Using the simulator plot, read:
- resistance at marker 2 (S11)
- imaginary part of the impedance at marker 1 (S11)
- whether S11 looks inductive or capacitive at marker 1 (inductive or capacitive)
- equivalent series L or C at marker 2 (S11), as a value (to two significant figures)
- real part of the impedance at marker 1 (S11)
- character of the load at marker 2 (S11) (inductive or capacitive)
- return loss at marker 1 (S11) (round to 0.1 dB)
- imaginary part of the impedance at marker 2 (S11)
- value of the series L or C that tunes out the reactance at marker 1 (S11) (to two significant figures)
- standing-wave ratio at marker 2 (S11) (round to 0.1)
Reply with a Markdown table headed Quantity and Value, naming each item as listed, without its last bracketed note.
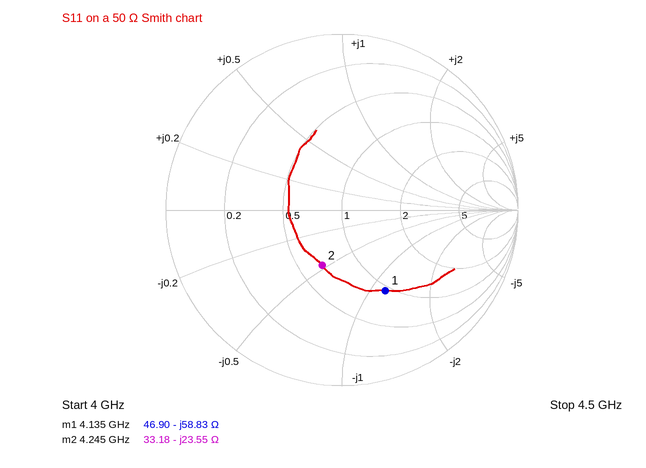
| Quantity | Value |
|---|---|
| resistance at marker 2 | 33.18 Ω |
| imaginary part of the impedance at marker 1 | -58.83 Ω |
| whether S11 looks inductive or capacitive at marker 1 | capacitive |
| equivalent series L or C at marker 2 (S11), as a value | 1.6 pF |
| real part of the impedance at marker 1 | 46.90 Ω |
| character of the load at marker 2 (S11) | capacitive |
| return loss at marker 1 (S11) | 5.7 dB |
| imaginary part of the impedance at marker 2 | -23.55 Ω |
| value of the series L or C that tunes out the reactance at marker 1 (S11) | 2.3 nH |
| standing-wave ratio at marker 2 (S11) | 2.0 |
